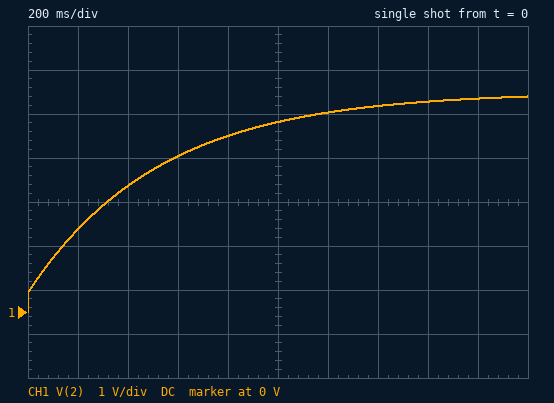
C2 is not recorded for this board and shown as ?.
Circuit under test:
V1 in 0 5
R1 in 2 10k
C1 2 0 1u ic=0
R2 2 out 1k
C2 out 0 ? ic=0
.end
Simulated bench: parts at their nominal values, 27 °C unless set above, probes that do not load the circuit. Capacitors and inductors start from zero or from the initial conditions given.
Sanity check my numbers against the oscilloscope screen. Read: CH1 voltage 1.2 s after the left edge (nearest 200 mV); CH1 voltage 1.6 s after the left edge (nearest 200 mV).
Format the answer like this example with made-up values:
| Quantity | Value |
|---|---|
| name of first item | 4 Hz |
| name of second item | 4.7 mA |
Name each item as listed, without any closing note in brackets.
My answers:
| Quantity | Value |
|---|---|
| CH1 voltage 1.2 s after the left edge | 4.6 V |
| CH1 voltage 1.6 s after the left edge | 4.8 V |
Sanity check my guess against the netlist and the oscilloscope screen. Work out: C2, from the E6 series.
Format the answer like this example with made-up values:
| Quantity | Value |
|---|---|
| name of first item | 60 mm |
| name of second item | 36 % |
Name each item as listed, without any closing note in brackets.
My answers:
| Quantity | Value |
|---|---|
| C2, from the E6 series | 47 µF |
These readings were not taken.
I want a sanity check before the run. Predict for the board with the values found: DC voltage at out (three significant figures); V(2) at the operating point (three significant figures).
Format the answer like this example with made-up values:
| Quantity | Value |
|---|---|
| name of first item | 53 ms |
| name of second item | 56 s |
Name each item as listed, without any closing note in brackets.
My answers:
| Quantity | Value |
|---|---|
| DC voltage at out | 5.00 V |
| V(2) at the operating point | 5.00 V |
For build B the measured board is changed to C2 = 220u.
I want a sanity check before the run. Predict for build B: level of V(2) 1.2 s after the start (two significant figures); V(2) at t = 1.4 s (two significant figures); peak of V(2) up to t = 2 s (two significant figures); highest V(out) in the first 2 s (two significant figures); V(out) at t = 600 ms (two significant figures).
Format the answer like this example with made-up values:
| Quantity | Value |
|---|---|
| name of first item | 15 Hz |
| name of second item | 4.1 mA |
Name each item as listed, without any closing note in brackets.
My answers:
| Quantity | Value |
|---|---|
| level of V(2) 1.2 s after the start | 2.2 V |
| V(2) at t = 1.4 s | 2.4 V |
| peak of V(2) up to t = 2 s | 3.0 V |
| highest V(out) in the first 2 s | 2.8 V |
| V(out) at t = 600 ms | 1.1 V |
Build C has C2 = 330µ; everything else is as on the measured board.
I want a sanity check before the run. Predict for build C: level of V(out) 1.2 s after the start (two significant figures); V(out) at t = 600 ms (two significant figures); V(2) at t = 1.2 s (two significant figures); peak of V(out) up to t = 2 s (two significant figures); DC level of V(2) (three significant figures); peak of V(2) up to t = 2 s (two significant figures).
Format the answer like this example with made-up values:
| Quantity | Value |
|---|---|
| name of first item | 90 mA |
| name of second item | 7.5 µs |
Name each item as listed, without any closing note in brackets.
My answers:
| Quantity | Value |
|---|---|
| level of V(out) 1.2 s after the start | 1.4 V |
| V(out) at t = 600 ms | 760 mV |
| V(2) at t = 1.2 s | 1.7 V |
| peak of V(out) up to t = 2 s | 2.1 V |
| DC level of V(2) | 5.00 V |
| peak of V(2) up to t = 2 s | 2.4 V |
